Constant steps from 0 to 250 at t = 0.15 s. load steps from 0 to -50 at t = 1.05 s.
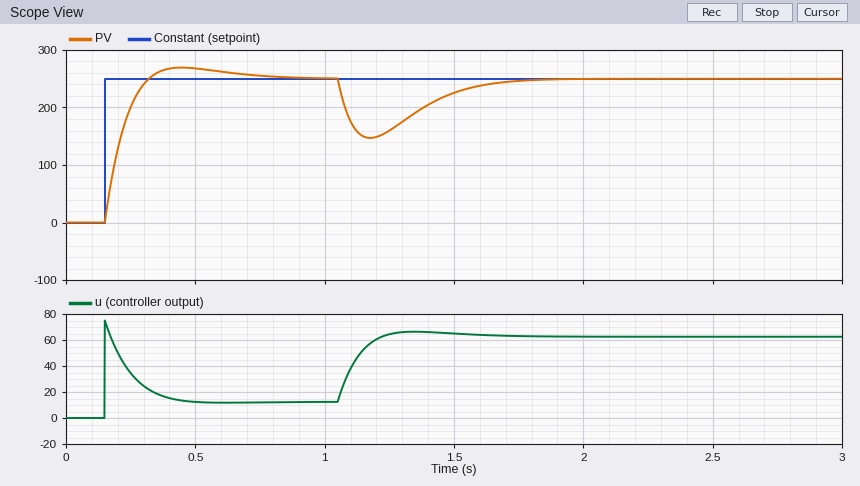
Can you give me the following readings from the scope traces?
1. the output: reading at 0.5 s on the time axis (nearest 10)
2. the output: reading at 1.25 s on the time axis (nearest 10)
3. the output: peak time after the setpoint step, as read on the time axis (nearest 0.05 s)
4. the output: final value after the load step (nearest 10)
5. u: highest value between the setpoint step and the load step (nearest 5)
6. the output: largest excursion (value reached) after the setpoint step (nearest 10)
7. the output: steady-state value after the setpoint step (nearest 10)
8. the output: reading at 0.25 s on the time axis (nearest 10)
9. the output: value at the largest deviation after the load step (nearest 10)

270
160
0.45 s
250
75
270
250
200
150
